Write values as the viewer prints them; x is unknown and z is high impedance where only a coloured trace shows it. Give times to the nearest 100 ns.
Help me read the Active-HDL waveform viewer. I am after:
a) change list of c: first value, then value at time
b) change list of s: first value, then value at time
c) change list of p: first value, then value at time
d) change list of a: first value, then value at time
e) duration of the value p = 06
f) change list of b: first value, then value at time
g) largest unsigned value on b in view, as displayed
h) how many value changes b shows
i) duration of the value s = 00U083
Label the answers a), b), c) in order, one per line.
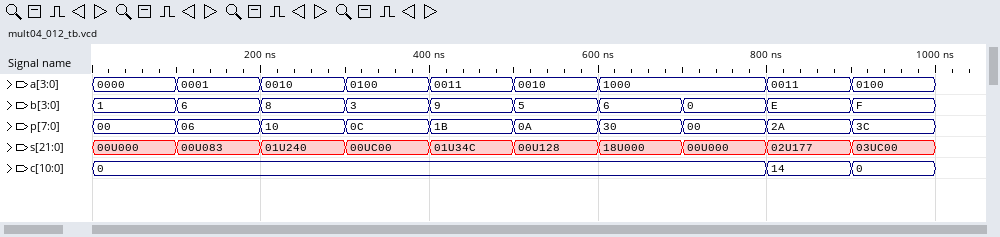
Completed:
a) 0, 14 at 800 ns, 0 at 900 ns
b) 00U000, 00U083 at 100 ns, 01U240 at 200 ns, 00UC00 at 300 ns, 01U34C at 400 ns, 00U128 at 500 ns, 18U000 at 600 ns, 00U000 at 700 ns, 02U177 at 800 ns, 03UC00 at 900 ns
c) 00, 06 at 100 ns, 10 at 200 ns, 0C at 300 ns, 1B at 400 ns, 0A at 500 ns, 30 at 600 ns, 00 at 700 ns, 2A at 800 ns, 3C at 900 ns
d) 0000, 0001 at 100 ns, 0010 at 200 ns, 0100 at 300 ns, 0011 at 400 ns, 0010 at 500 ns, 1000 at 600 ns, 0011 at 800 ns, 0100 at 900 ns
e) 100 ns
f) 1, 6 at 100 ns, 8 at 200 ns, 3 at 300 ns, 9 at 400 ns, 5 at 500 ns, 6 at 600 ns, 0 at 700 ns, E at 800 ns, F at 900 ns
g) F
h) 9
i) 100 ns
